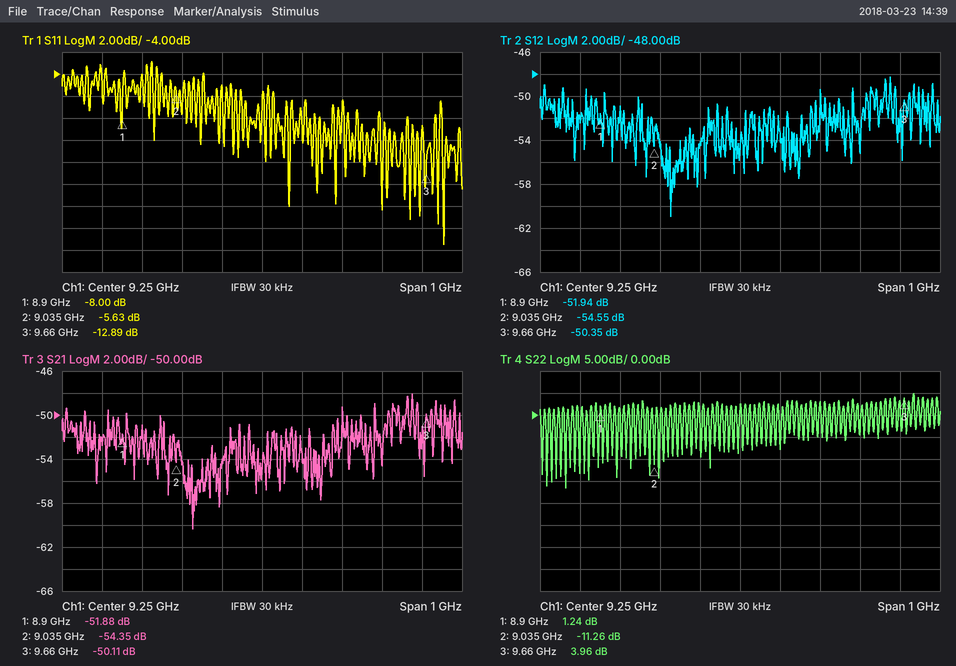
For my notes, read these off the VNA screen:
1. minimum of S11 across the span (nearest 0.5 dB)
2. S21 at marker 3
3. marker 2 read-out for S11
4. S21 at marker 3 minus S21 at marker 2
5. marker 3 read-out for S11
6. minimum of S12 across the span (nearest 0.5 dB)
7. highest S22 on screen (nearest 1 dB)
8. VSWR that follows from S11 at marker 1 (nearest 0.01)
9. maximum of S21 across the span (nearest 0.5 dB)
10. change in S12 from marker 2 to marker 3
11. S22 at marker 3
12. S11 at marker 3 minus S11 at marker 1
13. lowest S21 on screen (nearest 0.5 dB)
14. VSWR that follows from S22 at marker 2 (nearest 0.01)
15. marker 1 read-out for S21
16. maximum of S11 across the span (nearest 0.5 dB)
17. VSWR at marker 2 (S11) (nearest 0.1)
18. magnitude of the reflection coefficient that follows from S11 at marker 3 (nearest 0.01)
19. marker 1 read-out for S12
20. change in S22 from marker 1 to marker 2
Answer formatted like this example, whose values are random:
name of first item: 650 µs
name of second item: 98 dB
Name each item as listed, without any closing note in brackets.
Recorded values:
minimum of S11 across the span: -19.5 dB
S21 at marker 3: -50.11 dB
marker 2 read-out for S11: -5.63 dB
S21 at marker 3 minus S21 at marker 2: 4.24 dB
marker 3 read-out for S11: -12.89 dB
minimum of S12 across the span: -61.0 dB
highest S22 on screen: 5 dB
VSWR that follows from S11 at marker 1: 2.32
maximum of S21 across the span: -48.0 dB
change in S12 from marker 2 to marker 3: 4.20 dB
S22 at marker 3: 3.96 dB
S11 at marker 3 minus S11 at marker 1: -4.89 dB
lowest S21 on screen: -60.5 dB
VSWR that follows from S22 at marker 2: 1.75
marker 1 read-out for S21: -51.88 dB
maximum of S11 across the span: -3.0 dB
VSWR at marker 2 (S11): 3.2
magnitude of the reflection coefficient that follows from S11 at marker 3: 0.23
marker 1 read-out for S12: -51.94 dB
change in S22 from marker 1 to marker 2: -12.50 dB
